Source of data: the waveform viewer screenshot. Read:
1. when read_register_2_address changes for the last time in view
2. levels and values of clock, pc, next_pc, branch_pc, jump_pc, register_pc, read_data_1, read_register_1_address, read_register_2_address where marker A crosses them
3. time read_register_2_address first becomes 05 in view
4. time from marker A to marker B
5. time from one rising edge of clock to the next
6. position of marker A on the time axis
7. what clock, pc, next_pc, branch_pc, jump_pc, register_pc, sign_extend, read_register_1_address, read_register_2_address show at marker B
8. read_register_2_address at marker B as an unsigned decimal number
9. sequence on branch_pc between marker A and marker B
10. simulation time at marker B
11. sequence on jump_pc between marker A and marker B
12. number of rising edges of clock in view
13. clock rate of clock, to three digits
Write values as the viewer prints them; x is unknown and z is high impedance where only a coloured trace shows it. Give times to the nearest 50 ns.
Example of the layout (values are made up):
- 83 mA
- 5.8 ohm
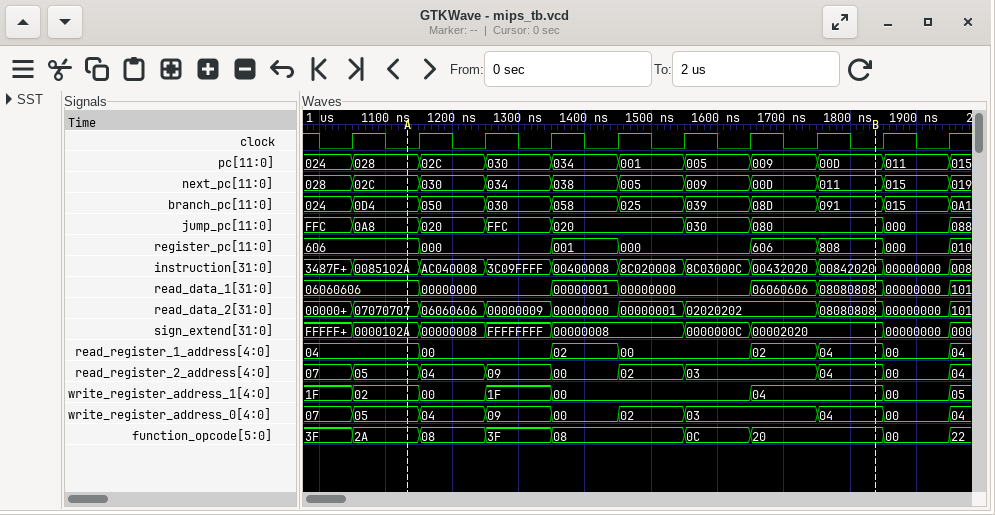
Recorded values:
- 1950 ns
- clock=0, pc=028, next_pc=02C, branch_pc=0D4, jump_pc=0A8, register_pc=606, read_data_1=06060606, read_register_1_address=04, read_register_2_address=05
- 1050 ns
- 700 ns
- 100 ns
- 1150 ns
- clock=0, pc=00D, next_pc=011, branch_pc=091, jump_pc=080, register_pc=808, sign_extend=00002020, read_register_1_address=04, read_register_2_address=04
- 4
- 0D4, 050, 030, 058, 025, 039, 08D, 091
- 1850 ns
- 0A8, 020, FFC, 020, 030, 080
- 10
- 10.0 MHz
